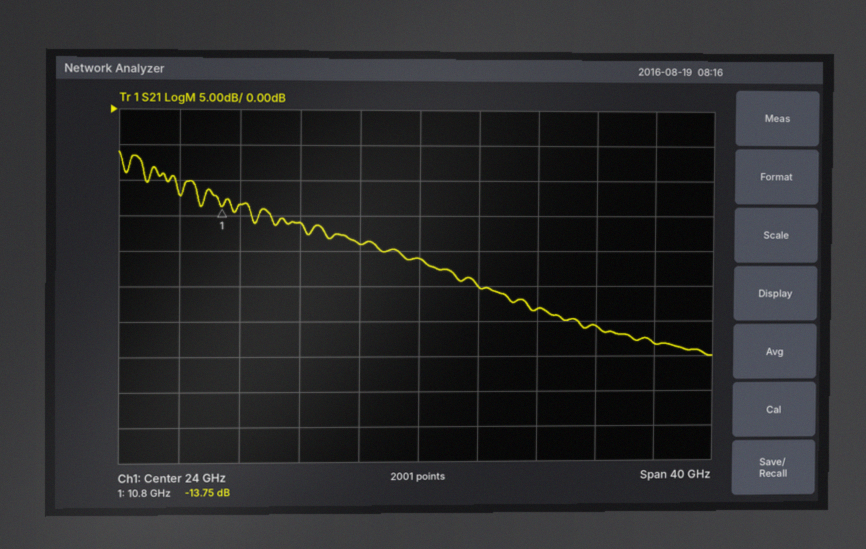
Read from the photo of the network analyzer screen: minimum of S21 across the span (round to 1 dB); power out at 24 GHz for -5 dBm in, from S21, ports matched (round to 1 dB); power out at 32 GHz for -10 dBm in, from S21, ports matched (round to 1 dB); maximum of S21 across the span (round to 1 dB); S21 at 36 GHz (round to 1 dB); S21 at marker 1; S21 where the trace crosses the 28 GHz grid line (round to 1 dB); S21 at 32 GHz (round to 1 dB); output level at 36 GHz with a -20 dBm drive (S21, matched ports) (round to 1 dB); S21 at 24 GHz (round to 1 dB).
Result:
-35 dB
-26 dBm
-38 dBm
-6 dB
-31 dB
-13.75 dB
-25 dB
-28 dB
-51 dBm
-21 dB
